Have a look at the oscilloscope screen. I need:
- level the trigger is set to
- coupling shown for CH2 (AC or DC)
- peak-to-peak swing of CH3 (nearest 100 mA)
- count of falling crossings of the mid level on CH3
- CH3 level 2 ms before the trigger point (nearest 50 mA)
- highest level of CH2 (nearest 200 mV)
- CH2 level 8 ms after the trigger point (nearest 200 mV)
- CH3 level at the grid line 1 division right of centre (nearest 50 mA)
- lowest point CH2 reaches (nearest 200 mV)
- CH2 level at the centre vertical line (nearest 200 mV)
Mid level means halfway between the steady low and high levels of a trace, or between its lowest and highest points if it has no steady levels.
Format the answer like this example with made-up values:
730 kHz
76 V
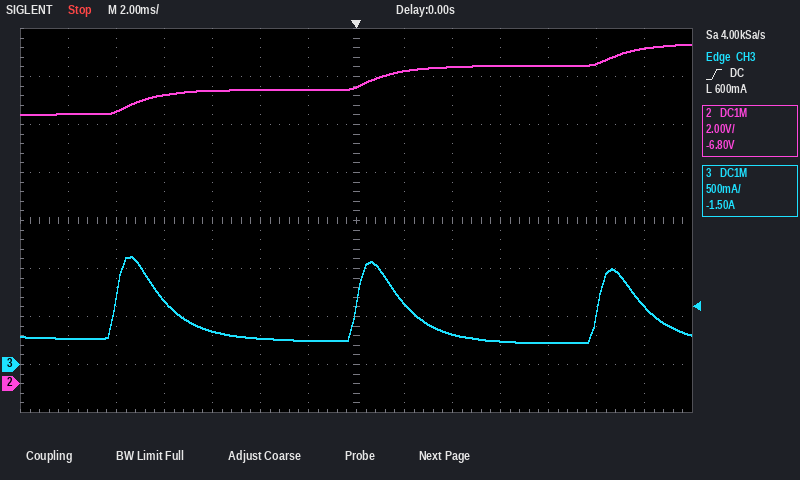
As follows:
600 mA
DC
900 mA
3
250 mA
14.2 V
13.2 V
650 mA
11.2 V
12.4 V
